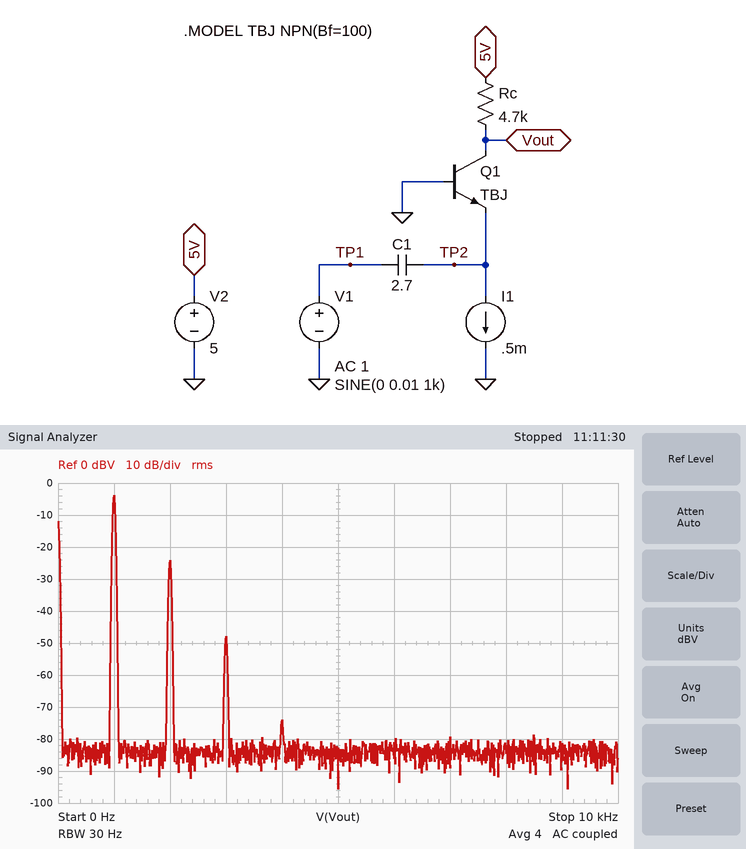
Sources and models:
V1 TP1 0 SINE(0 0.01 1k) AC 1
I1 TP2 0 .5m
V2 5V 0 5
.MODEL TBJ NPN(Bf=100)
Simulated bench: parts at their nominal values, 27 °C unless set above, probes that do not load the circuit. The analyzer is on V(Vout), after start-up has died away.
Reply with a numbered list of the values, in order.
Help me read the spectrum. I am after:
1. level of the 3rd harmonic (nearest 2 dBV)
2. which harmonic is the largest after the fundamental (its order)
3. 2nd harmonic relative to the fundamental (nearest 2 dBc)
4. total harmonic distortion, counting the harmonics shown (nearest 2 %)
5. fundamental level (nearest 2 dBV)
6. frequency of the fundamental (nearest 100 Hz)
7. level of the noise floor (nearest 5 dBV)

1. -48 dBV
2. 2
3. -20 dBc
4. 10 %
5. -4 dBV
6. 1.0 kHz
7. -85 dBV
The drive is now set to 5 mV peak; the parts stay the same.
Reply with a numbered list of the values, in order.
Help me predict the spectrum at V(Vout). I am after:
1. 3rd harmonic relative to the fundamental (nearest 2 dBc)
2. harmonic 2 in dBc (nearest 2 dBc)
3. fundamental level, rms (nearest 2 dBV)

1. -56 dBc
2. -26 dBc
3. -10 dBV
